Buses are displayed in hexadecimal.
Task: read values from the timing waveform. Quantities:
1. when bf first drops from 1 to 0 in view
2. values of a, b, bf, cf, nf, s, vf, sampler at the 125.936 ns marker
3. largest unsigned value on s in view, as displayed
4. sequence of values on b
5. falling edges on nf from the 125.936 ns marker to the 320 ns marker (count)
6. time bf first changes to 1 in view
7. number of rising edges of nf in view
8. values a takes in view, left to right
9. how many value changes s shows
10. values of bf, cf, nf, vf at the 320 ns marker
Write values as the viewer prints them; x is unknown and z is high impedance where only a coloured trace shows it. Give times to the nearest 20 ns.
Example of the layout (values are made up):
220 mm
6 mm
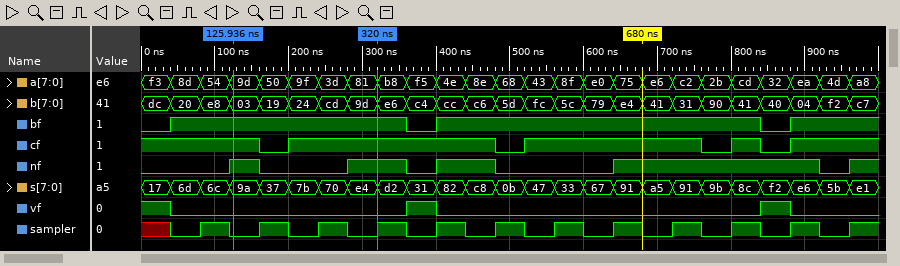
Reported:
360 ns
a=9d, b=03, bf=1, cf=1, nf=1, s=9a, vf=0, sampler=0
f2
dc, 20, e8, 03, 19, 24, cd, 9d, e6, c4, cc, c6, 5d, fc, 5c, 79, e4, 41, 31, 90, 41, 40, 04, f2, c7
1
40 ns
5
f3, 8d, 54, 9d, 50, 9f, 3d, 81, b8, f5, 4e, 8e, 68, 43, 8f, e0, 75, e6, c2, 2b, cd, 32, ea, 4d, a8
24
bf=1, cf=1, nf=1, vf=0
